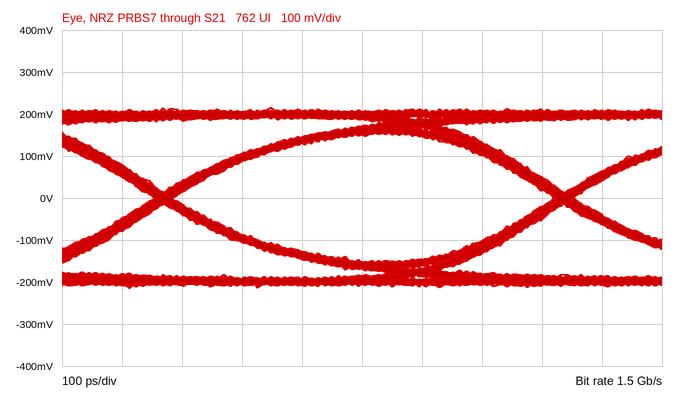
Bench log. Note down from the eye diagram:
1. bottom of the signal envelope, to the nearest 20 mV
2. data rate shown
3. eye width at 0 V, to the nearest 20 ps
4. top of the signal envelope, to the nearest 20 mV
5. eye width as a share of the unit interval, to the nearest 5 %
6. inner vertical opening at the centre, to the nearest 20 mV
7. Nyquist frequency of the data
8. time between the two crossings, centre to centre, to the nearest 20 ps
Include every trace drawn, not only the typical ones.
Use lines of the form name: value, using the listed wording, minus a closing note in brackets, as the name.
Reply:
bottom of the signal envelope, to the nearest 20 mV: -220 mV
data rate shown: 1.5 Gb/s
eye width at 0 V, to the nearest 20 ps: 640 ps
top of the signal envelope, to the nearest 20 mV: 220 mV
eye width as a share of the unit interval, to the nearest 5 %: 95 %
inner vertical opening at the centre, to the nearest 20 mV: 300 mV
Nyquist frequency of the data: 750 MHz
time between the two crossings, centre to centre, to the nearest 20 ps: 660 ps
